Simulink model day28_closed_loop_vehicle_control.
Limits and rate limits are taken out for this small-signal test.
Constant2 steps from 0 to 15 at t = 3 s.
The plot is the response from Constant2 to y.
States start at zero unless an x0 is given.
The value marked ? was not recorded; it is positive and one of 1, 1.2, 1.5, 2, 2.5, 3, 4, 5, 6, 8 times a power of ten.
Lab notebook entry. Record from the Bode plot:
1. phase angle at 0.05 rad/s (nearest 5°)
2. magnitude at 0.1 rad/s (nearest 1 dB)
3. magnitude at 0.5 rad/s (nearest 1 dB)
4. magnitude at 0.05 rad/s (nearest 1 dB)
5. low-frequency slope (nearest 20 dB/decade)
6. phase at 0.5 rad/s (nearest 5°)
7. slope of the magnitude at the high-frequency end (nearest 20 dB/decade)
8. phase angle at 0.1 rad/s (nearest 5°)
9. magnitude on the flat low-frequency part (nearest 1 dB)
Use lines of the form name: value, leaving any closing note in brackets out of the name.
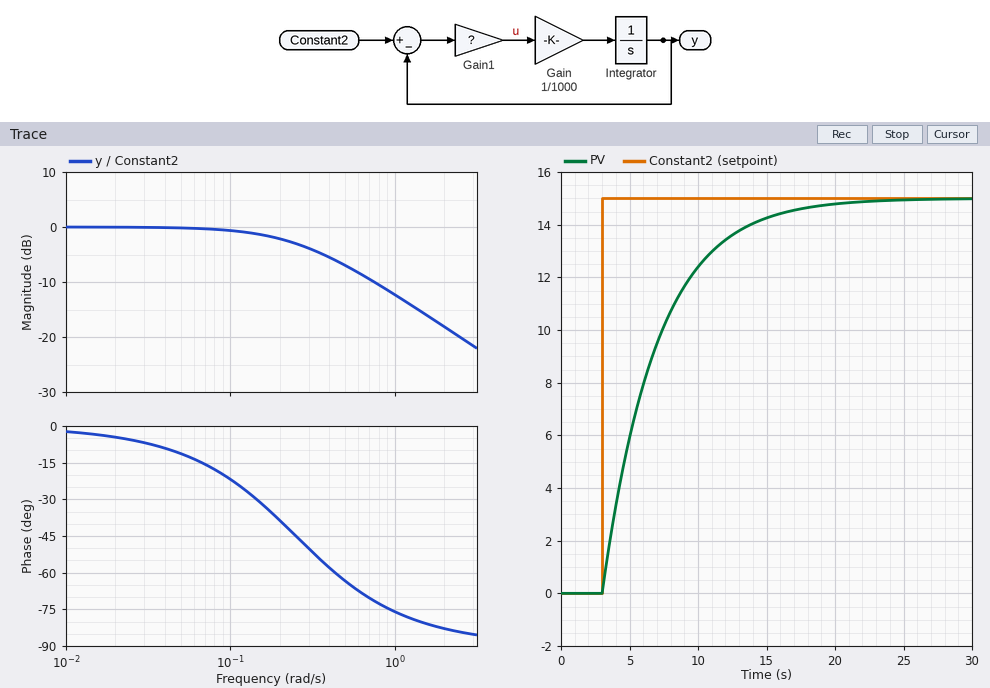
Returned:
phase angle at 0.05 rad/s: -10°
magnitude at 0.1 rad/s: -1 dB
magnitude at 0.5 rad/s: -7 dB
magnitude at 0.05 rad/s: 0 dB
low-frequency slope: 0 dB/decade
phase at 0.5 rad/s: -65°
slope of the magnitude at the high-frequency end: -20 dB/decade
phase angle at 0.1 rad/s: -20°
magnitude on the flat low-frequency part: 0 dB
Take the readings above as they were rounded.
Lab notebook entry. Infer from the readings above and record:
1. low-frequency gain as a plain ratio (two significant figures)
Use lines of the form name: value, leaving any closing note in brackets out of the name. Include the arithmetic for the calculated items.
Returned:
low-frequency gain as a plain ratio: 10^(0 / 20) = 1.0
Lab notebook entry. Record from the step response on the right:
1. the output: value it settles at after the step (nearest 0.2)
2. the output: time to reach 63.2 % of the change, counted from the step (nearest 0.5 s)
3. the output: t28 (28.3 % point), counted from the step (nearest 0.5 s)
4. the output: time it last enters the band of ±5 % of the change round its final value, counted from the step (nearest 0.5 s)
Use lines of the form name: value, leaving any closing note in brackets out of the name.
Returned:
the output: value it settles at after the step: 15.0
the output: time to reach 63.2 % of the change, counted from the step: 4.0 s
the output: t28 (28.3 % point), counted from the step: 1.5 s
the output: time it last enters the band of ±5 % of the change round its final value, counted from the step: 12.0 s
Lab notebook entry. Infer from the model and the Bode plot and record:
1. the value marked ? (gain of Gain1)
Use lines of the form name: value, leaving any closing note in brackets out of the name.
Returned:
the value marked ?: 250
